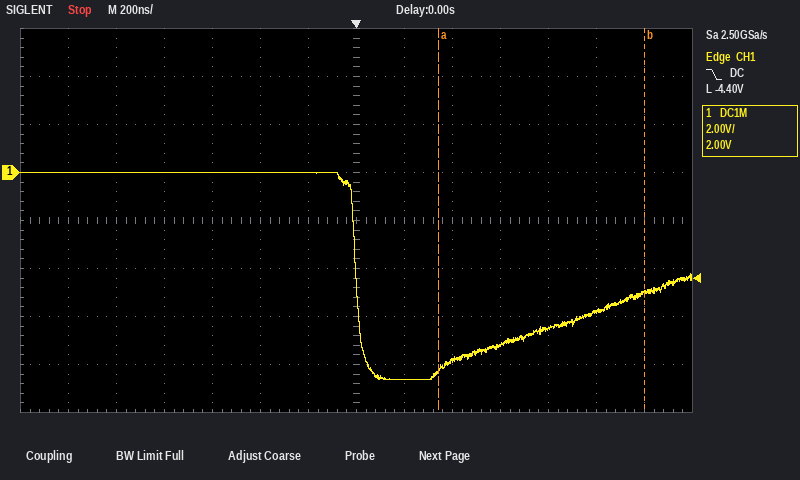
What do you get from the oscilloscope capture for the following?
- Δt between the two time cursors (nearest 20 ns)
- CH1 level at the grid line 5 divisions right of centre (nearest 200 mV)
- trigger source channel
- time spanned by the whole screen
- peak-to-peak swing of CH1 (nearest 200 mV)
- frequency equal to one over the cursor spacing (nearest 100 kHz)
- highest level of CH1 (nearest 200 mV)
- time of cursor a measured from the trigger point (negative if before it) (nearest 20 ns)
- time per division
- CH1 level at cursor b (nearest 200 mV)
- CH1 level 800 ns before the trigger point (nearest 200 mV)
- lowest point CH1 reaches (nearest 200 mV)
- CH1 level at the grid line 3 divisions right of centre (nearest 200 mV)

860 ns
-5.8 V
CH1
2.8 µs
8.6 V
1.2 MHz
0.0 V
+340 ns
200 ns
-5.0 V
0.0 V
-8.6 V
-7.2 V
